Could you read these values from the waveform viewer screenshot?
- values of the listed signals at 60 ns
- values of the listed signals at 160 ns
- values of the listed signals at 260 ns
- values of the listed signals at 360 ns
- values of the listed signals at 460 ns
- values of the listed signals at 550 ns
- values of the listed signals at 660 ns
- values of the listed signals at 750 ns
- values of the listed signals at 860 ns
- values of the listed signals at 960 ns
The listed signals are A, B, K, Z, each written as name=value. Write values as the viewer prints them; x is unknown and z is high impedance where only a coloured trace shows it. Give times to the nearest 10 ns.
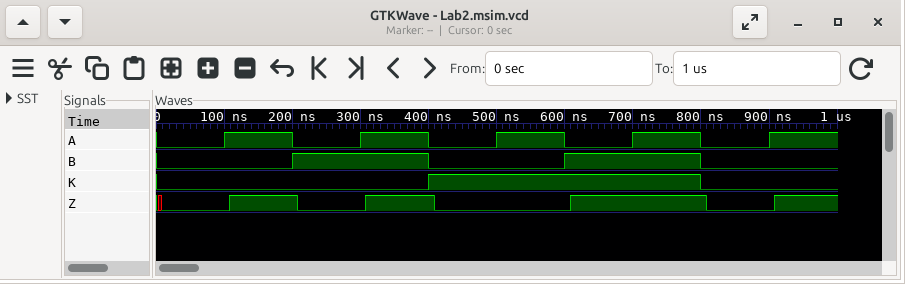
A=0, B=0, K=0, Z=0
A=1, B=0, K=0, Z=1
A=0, B=1, K=0, Z=0
A=1, B=1, K=0, Z=1
A=0, B=0, K=1, Z=0
A=1, B=0, K=1, Z=0
A=0, B=1, K=1, Z=1
A=1, B=1, K=1, Z=1
A=0, B=0, K=0, Z=0
A=1, B=0, K=0, Z=1
